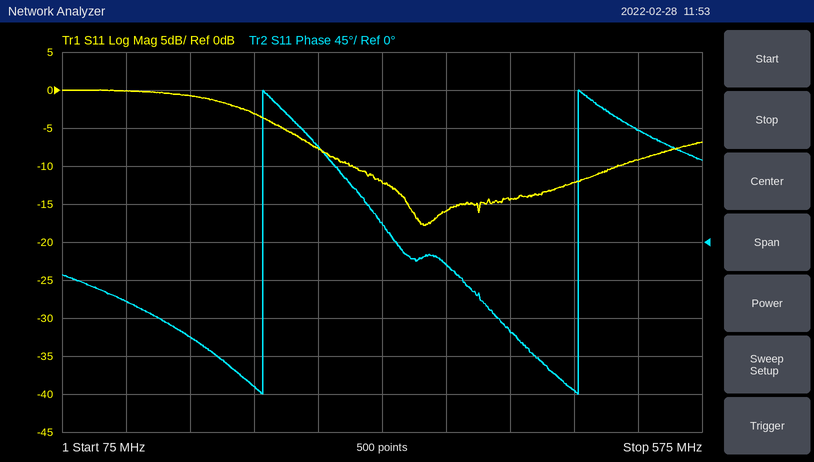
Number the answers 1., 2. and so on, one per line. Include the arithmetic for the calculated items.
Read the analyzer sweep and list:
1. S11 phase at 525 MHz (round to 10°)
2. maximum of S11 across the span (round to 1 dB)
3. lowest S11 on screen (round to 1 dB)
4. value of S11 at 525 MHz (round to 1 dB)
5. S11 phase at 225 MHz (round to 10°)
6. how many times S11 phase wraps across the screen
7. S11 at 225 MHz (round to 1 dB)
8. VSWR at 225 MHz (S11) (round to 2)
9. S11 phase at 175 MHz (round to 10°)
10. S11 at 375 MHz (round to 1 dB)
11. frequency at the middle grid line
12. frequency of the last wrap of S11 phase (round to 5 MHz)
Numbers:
1. 130°
2. 0 dB
3. -18 dB
4. -9 dB
5. -170°
6. 2
7. -3 dB
8. |Γ| = 10^(-3/20) = 0.7079; VSWR = (1 + 0.7079)/(1 − 0.7079) ≈ 6
9. -110°
10. -16 dB
11. 325 MHz
12. 480 MHz
